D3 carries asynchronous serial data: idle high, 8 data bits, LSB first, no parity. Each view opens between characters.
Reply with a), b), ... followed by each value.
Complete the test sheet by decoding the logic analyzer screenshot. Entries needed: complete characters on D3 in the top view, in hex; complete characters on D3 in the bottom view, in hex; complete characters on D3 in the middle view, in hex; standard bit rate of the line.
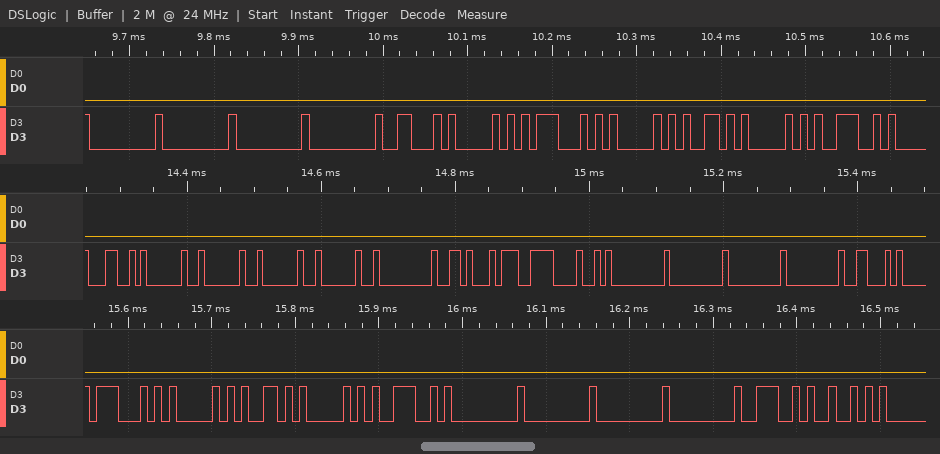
a) 00, 00, 00, 00, 46, 50, 47, 41, 59, 50, 4E
b) 47, 41, 59, 50, 4E, 00, 00, 00, 00, 4E, 52
c) 4C, 20, 20, 20, 20, 00, 16, E7, 48, 00, 00, 00, 00, 46
d) 115200 baud
